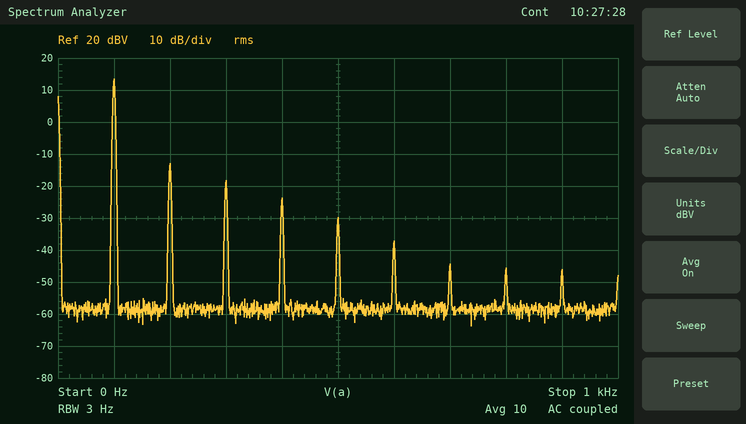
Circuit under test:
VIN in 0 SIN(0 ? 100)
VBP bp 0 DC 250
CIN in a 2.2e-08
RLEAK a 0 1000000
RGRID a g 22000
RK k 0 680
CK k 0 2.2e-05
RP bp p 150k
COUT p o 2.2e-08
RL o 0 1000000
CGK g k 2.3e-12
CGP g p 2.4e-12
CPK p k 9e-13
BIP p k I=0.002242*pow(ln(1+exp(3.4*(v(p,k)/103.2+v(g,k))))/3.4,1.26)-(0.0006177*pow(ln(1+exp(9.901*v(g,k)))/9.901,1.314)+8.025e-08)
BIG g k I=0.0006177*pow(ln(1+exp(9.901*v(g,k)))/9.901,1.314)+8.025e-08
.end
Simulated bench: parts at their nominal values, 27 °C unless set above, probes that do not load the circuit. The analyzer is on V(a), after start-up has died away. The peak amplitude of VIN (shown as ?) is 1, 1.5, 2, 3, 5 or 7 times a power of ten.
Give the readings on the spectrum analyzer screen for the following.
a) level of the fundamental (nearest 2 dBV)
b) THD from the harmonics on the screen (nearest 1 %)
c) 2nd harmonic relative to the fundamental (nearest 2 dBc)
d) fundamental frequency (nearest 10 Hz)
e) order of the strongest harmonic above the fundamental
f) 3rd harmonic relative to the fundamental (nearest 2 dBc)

14 dBV
6 %
-26 dBc
100 Hz
2
-32 dBc
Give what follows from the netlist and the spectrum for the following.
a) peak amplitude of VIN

7 V
